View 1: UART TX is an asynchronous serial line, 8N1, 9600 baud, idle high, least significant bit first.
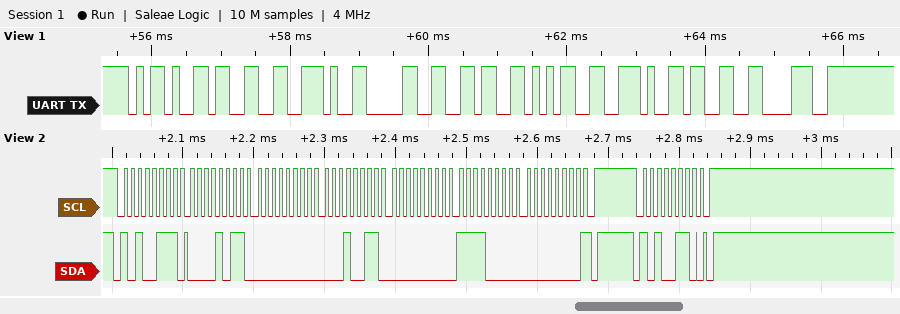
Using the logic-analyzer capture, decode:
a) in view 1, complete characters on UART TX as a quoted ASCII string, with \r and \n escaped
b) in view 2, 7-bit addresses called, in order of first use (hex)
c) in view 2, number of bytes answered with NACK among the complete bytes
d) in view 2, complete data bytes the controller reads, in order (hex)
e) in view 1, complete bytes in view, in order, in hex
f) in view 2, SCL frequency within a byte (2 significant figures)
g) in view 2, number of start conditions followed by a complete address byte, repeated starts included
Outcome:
"-3.065.38"
0x53
1
0B 00 13 00 F0 00
2D 33 2E 30 36 35 2E 33 38
100 kHz
2
